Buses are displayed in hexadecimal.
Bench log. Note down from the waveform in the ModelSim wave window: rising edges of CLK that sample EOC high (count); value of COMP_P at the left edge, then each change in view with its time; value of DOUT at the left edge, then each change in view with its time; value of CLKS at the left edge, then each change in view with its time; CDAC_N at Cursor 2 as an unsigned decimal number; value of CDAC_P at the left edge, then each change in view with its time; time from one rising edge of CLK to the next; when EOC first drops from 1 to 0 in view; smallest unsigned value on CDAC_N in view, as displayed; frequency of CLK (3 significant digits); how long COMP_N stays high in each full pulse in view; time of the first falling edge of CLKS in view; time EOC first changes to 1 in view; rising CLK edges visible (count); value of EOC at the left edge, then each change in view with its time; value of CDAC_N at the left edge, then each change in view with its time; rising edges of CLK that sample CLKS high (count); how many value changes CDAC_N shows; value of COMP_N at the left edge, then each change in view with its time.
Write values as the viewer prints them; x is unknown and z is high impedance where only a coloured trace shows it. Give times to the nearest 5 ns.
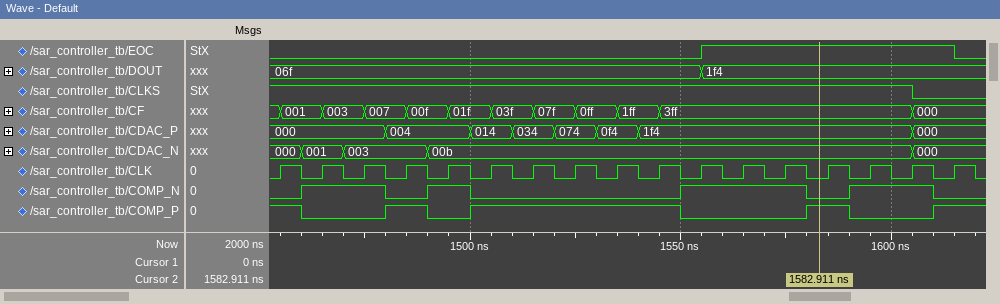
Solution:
6
1, 0 at 1460 ns, 1 at 1480 ns, 0 at 1490 ns, 1 at 1500 ns, 0 at 1550 ns, 1 at 1580 ns, 0 at 1590 ns, 1 at 1610 ns
06f, 1f4 at 1555 ns
1, 0 at 1605 ns
11
000, 004 at 1480 ns, 014 at 1500 ns, 034 at 1510 ns, 074 at 1520 ns, 0f4 at 1530 ns, 1f4 at 1540 ns, 000 at 1605 ns
10 ns
1615 ns
000
100 MHz
20 ns, 10 ns, 30 ns, 20 ns
1605 ns
1555 ns
17
0, 1 at 1555 ns, 0 at 1615 ns
000, 001 at 1460 ns, 003 at 1470 ns, 00b at 1490 ns, 000 at 1605 ns
16
4
0, 1 at 1460 ns, 0 at 1480 ns, 1 at 1490 ns, 0 at 1500 ns, 1 at 1550 ns, 0 at 1580 ns, 1 at 1590 ns, 0 at 1610 ns
